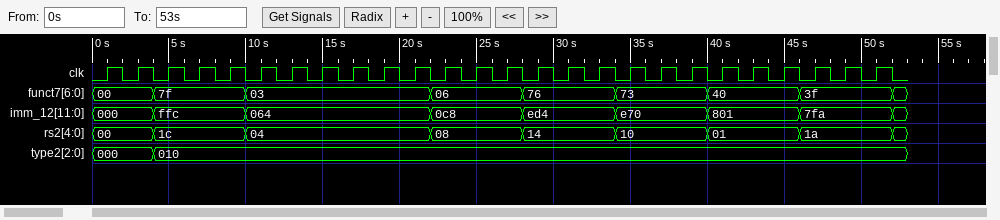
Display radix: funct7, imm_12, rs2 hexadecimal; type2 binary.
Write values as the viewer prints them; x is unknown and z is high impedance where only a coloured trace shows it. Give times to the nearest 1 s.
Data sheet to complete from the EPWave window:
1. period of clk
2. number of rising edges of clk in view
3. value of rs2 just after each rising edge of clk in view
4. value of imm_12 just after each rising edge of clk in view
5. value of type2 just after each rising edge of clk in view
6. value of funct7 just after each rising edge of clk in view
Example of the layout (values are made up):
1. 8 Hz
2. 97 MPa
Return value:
1. 2 s
2. 26
3. 00, 00, 1c, 1c, 1c, 04, 04, 04, 04, 04, 04, 08, 08, 08, 14, 14, 14, 10, 10, 10, 01, 01, 01, 1a, 1a, 1a
4. 000, 000, ffc, ffc, ffc, 064, 064, 064, 064, 064, 064, 0c8, 0c8, 0c8, ed4, ed4, ed4, e70, e70, e70, 801, 801, 801, 7fa, 7fa, 7fa
5. 000, 000, 010, 010, 010, 010, 010, 010, 010, 010, 010, 010, 010, 010, 010, 010, 010, 010, 010, 010, 010, 010, 010, 010, 010, 010
6. 00, 00, 7f, 7f, 7f, 03, 03, 03, 03, 03, 03, 06, 06, 06, 76, 76, 76, 73, 73, 73, 40, 40, 40, 3f, 3f, 3f
